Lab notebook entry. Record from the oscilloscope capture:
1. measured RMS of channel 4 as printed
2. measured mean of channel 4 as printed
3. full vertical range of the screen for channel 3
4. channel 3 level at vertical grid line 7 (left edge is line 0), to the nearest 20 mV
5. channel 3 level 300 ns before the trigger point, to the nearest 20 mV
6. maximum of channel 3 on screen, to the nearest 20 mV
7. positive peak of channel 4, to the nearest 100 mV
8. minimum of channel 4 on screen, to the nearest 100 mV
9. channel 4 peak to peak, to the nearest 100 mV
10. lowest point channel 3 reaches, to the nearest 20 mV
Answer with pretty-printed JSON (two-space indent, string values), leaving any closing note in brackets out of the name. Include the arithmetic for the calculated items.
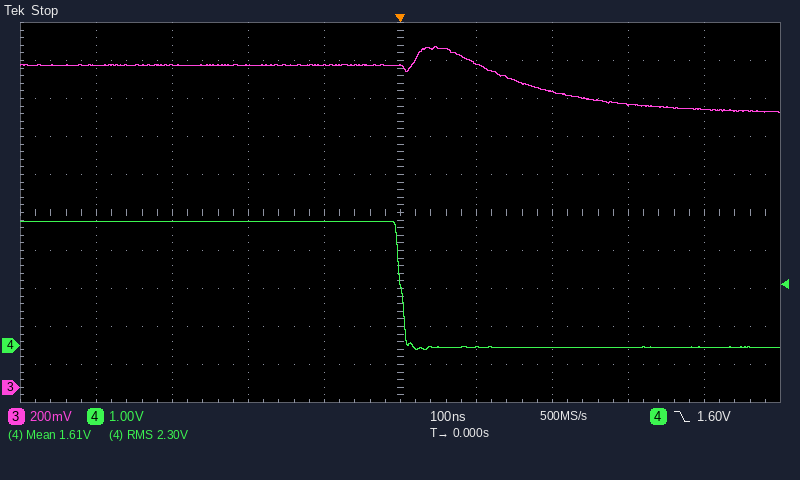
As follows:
{
  "measured RMS of channel 4 as printed": "2.30 V",
  "measured mean of channel 4 as printed": "1.61 V",
  "full vertical range of the screen for channel 3": "2 V",
  "channel 3 level at vertical grid line 7 (left edge is line 0), to the nearest 20 mV": "1.56 V",
  "channel 3 level 300 ns before the trigger point, to the nearest 20 mV": "1.70 V",
  "maximum of channel 3 on screen, to the nearest 20 mV": "1.80 V",
  "positive peak of channel 4, to the nearest 100 mV": "3.3 V",
  "minimum of channel 4 on screen, to the nearest 100 mV": "-100 mV",
  "channel 4 peak to peak, to the nearest 100 mV": "3.3 V − (-100 mV) = 3.4 V",
  "lowest point channel 3 reaches, to the nearest 20 mV": "1.44 V"
}
